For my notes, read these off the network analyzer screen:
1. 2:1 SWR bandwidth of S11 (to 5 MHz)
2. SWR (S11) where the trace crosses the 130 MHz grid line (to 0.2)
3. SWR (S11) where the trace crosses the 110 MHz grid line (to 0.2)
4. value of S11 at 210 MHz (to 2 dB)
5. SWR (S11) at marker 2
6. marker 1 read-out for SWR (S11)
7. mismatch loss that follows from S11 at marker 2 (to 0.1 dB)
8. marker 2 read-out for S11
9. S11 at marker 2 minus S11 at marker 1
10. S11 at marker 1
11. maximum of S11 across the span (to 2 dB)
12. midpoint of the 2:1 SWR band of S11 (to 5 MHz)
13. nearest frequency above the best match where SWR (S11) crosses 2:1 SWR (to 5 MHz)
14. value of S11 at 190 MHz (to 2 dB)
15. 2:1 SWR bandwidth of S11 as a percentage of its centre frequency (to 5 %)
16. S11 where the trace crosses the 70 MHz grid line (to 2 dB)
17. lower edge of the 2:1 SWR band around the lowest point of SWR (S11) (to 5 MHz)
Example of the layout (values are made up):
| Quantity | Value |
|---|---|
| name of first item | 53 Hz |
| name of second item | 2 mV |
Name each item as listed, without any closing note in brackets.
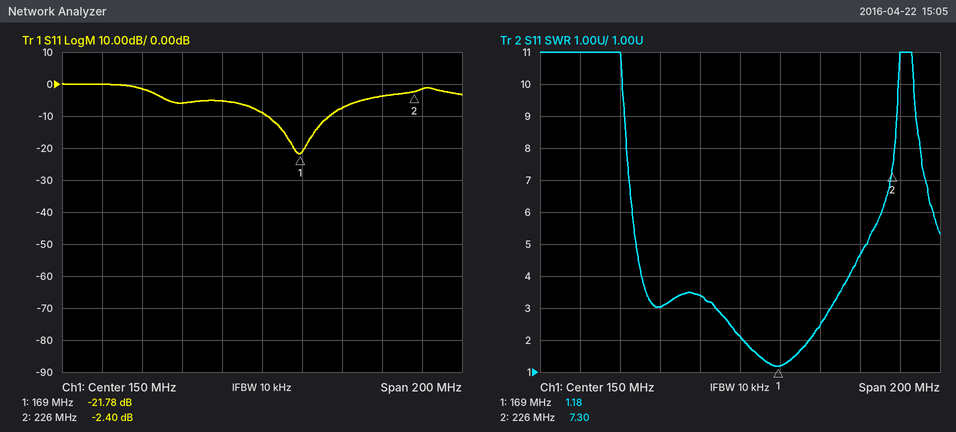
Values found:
| Quantity | Value |
|---|---|
| 2:1 SWR bandwidth of S11 | 35 MHz |
| SWR (S11) where the trace crosses the 130 MHz grid line | 3.4 |
| SWR (S11) where the trace crosses the 110 MHz grid line | 3.0 |
| value of S11 at 210 MHz | -4 dB |
| SWR (S11) at marker 2 | 7.30 |
| marker 1 read-out for SWR | 1.18 |
| mismatch loss that follows from S11 at marker 2 | 3.7 dB |
| marker 2 read-out for S11 | -2.40 dB |
| S11 at marker 2 minus S11 at marker 1 | 19.38 dB |
| S11 at marker 1 | -21.78 dB |
| maximum of S11 across the span | 0 dB |
| midpoint of the 2:1 SWR band of S11 | 170 MHz |
| nearest frequency above the best match where SWR (S11) crosses 2:1 SWR | 185 MHz |
| value of S11 at 190 MHz | -8 dB |
| 2:1 SWR bandwidth of S11 as a percentage of its centre frequency | 20 % |
| S11 where the trace crosses the 70 MHz grid line | 0 dB |
| lower edge of the 2:1 SWR band around the lowest point of SWR (S11) | 150 MHz |
